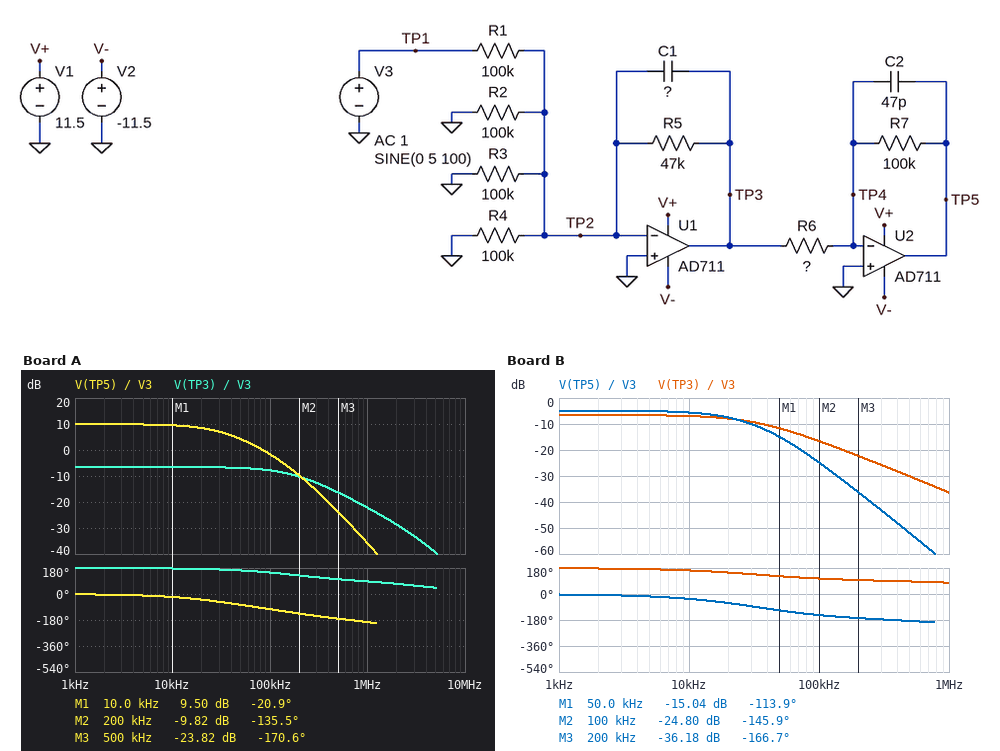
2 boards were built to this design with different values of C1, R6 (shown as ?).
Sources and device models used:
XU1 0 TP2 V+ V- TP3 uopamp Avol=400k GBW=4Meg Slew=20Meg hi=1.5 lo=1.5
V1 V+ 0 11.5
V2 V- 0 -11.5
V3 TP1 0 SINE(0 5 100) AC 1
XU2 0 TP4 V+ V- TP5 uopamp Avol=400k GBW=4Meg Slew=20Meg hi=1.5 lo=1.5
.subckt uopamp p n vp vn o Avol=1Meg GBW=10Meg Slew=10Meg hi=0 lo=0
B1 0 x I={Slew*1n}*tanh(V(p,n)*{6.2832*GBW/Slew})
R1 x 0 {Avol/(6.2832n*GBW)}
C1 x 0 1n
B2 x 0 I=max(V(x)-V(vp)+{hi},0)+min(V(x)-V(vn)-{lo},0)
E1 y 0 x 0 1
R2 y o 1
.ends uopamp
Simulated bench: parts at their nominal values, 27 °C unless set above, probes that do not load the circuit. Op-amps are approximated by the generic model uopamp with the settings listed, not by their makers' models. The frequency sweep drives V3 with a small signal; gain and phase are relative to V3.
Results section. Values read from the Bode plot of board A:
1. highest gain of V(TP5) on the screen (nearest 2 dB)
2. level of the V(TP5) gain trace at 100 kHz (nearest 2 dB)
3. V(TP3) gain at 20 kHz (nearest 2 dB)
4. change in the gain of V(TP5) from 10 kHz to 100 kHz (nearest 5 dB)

10 dB
-2 dB
-6 dB
-10 dB
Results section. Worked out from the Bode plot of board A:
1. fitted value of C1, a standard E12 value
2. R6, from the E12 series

18 pF
15 kΩ
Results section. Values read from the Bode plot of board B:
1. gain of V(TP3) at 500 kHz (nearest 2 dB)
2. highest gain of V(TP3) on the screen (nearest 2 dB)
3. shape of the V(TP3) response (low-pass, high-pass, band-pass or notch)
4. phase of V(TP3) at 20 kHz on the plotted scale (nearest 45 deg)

-30 dB
-6 dB
low-pass
135 deg
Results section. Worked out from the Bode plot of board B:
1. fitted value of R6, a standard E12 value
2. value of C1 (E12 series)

82 kΩ
100 pF
